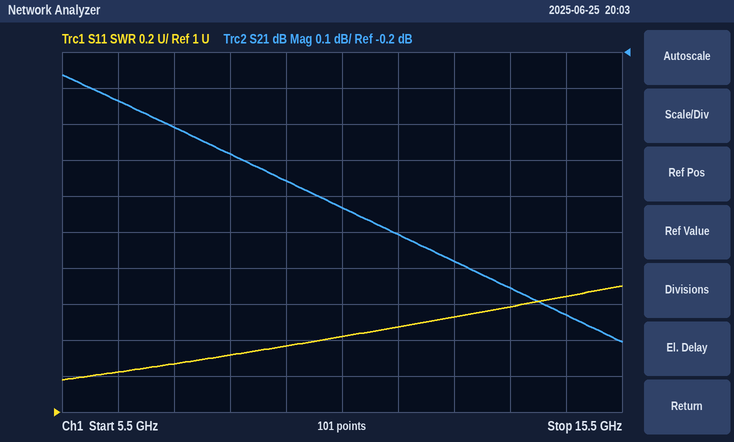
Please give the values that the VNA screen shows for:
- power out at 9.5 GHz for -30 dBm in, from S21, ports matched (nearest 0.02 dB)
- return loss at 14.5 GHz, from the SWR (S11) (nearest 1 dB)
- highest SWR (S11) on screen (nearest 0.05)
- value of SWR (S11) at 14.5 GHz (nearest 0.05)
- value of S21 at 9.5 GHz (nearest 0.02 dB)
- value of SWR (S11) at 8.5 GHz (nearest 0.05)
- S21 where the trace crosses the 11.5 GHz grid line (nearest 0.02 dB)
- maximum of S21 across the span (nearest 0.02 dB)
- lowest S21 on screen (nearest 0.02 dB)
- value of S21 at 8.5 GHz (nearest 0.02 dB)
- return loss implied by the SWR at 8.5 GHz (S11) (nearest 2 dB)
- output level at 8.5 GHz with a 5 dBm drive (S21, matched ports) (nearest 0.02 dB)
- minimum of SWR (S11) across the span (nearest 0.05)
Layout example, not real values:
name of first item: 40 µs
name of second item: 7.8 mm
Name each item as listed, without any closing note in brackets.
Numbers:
power out at 9.5 GHz for -30 dBm in, from S21, ports matched: -30.56 dBm
return loss at 14.5 GHz, from the SWR (S11): 12 dB
highest SWR (S11) on screen: 1.70
value of SWR (S11) at 14.5 GHz: 1.65
value of S21 at 9.5 GHz: -0.56 dB
value of SWR (S11) at 8.5 GHz: 1.30
S21 where the trace crosses the 11.5 GHz grid line: -0.70 dB
maximum of S21 across the span: -0.26 dB
lowest S21 on screen: -1.00 dB
value of S21 at 8.5 GHz: -0.48 dB
return loss implied by the SWR at 8.5 GHz (S11): 18 dB
output level at 8.5 GHz with a 5 dBm drive (S21, matched ports): 4.52 dBm
minimum of SWR (S11) across the span: 1.20
